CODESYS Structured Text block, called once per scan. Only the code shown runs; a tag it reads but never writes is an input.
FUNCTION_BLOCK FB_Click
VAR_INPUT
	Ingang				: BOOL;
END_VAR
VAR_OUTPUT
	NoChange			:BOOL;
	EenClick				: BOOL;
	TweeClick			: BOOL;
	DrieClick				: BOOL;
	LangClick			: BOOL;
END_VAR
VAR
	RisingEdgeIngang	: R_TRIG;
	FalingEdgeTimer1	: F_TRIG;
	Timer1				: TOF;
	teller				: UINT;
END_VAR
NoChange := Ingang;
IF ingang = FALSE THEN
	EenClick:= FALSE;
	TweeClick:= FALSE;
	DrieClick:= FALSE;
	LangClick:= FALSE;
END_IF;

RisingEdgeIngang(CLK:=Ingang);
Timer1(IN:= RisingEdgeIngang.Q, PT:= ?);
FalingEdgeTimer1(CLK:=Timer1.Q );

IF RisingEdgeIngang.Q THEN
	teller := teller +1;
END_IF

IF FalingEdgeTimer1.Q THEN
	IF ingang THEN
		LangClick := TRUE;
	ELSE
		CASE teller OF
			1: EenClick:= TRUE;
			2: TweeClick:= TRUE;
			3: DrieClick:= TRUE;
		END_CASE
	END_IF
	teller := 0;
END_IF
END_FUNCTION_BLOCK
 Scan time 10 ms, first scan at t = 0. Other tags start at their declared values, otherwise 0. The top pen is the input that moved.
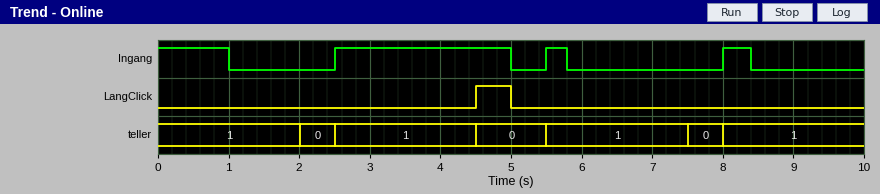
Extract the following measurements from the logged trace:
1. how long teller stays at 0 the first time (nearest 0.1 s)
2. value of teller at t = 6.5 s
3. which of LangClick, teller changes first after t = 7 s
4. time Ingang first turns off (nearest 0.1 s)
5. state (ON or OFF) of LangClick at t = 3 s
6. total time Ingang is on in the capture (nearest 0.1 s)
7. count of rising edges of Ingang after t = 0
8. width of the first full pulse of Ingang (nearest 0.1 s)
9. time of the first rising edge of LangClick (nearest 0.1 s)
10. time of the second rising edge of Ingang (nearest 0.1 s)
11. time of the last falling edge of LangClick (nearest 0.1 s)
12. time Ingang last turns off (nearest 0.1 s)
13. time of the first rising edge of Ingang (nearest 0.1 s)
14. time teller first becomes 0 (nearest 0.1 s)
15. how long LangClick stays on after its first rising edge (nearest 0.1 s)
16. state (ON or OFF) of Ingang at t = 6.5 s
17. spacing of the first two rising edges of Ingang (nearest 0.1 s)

0.5 s
1
teller
1.0 s
OFF
4.2 s
3
2.5 s
4.5 s
5.5 s
5.0 s
8.4 s
2.5 s
2.0 s
0.5 s
OFF
3.0 s
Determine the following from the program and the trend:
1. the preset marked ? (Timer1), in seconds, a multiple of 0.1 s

2.0 s
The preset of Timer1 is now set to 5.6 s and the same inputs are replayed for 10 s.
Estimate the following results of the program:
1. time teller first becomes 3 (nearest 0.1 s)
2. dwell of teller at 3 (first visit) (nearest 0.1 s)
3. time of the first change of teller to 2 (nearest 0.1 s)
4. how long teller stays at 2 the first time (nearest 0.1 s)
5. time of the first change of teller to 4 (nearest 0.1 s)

5.5 s
2.5 s
2.5 s
3.0 s
8.0 s
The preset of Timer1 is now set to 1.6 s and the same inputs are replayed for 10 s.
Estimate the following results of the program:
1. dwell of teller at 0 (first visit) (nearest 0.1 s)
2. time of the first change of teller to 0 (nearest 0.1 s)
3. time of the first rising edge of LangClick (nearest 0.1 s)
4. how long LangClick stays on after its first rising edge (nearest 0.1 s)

0.9 s
1.6 s
4.1 s
0.9 s
